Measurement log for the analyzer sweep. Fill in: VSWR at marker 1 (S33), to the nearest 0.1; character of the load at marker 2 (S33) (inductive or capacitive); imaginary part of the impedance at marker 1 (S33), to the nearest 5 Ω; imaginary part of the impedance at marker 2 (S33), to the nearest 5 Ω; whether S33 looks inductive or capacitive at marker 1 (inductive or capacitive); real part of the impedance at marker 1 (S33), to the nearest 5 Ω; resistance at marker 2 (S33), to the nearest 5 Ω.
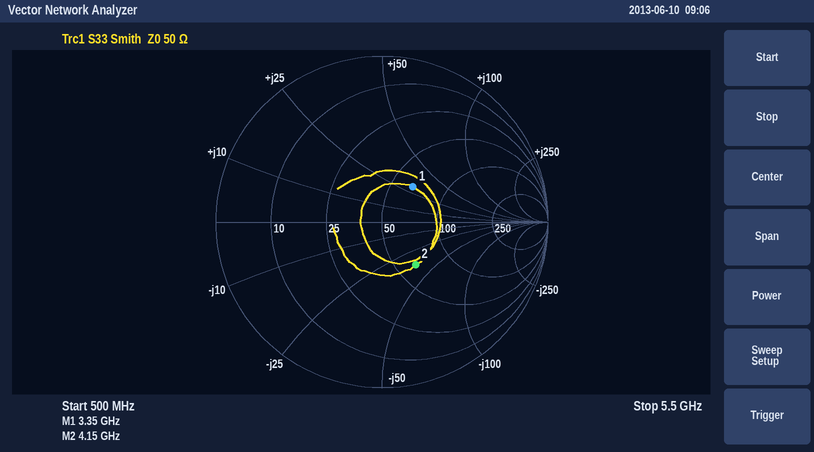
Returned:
1.8
capacitive
+30 Ω
-35 Ω
inductive
65 Ω
65 Ω
